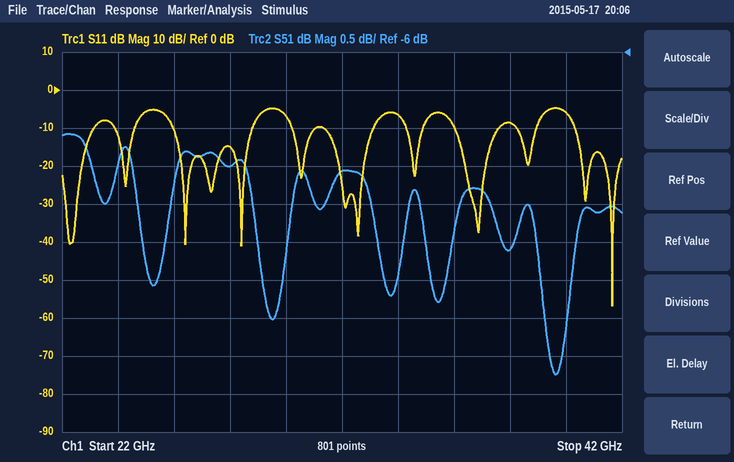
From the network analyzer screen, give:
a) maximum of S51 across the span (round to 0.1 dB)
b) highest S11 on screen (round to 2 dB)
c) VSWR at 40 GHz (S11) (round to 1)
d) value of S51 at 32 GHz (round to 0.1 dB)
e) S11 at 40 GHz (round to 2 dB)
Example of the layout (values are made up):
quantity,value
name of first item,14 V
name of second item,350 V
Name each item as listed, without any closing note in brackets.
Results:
quantity,value
maximum of S51 across the span,-7.1 dB
highest S11 on screen,-4 dB
VSWR at 40 GHz (S11),3
value of S51 at 32 GHz,-7.6 dB
S11 at 40 GHz,-6 dB
